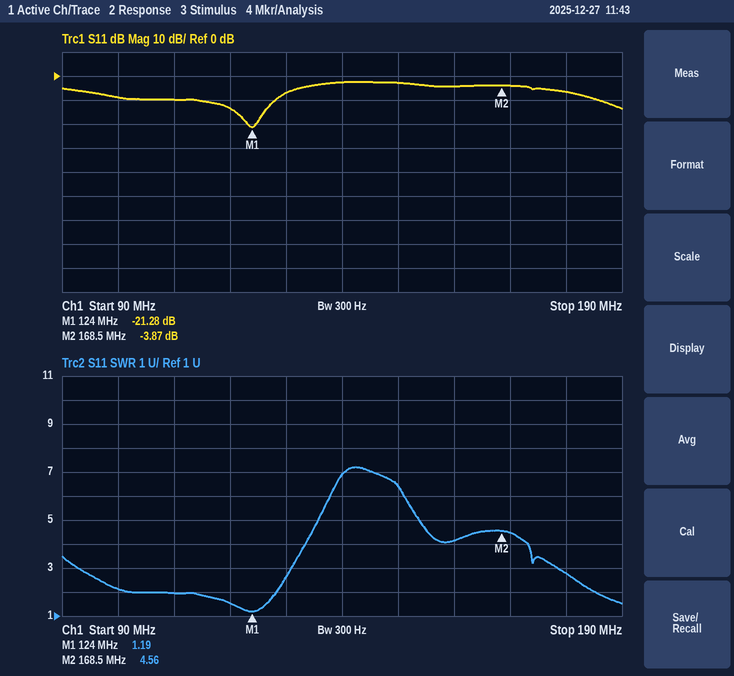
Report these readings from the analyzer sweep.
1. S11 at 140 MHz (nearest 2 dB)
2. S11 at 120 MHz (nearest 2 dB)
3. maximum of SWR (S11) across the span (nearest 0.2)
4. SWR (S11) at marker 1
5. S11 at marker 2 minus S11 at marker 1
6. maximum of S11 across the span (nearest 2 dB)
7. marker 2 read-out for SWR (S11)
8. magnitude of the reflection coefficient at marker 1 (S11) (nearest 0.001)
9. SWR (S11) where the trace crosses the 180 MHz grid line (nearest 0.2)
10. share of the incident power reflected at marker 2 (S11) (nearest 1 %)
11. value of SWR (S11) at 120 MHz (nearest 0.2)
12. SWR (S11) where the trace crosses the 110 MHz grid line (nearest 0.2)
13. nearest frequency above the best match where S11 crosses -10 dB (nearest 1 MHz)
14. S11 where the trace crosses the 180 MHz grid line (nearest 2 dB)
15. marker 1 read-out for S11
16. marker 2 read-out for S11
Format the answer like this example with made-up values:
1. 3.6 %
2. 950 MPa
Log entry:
1. -2 dB
2. -14 dB
3. 7.2
4. 1.19
5. 17.41 dB
6. -2 dB
7. 4.56
8. 0.086
9. 2.8
10. 41 %
11. 1.6
12. 2.0
13. 128 MHz
14. -6 dB
15. -21.28 dB
16. -3.87 dB
